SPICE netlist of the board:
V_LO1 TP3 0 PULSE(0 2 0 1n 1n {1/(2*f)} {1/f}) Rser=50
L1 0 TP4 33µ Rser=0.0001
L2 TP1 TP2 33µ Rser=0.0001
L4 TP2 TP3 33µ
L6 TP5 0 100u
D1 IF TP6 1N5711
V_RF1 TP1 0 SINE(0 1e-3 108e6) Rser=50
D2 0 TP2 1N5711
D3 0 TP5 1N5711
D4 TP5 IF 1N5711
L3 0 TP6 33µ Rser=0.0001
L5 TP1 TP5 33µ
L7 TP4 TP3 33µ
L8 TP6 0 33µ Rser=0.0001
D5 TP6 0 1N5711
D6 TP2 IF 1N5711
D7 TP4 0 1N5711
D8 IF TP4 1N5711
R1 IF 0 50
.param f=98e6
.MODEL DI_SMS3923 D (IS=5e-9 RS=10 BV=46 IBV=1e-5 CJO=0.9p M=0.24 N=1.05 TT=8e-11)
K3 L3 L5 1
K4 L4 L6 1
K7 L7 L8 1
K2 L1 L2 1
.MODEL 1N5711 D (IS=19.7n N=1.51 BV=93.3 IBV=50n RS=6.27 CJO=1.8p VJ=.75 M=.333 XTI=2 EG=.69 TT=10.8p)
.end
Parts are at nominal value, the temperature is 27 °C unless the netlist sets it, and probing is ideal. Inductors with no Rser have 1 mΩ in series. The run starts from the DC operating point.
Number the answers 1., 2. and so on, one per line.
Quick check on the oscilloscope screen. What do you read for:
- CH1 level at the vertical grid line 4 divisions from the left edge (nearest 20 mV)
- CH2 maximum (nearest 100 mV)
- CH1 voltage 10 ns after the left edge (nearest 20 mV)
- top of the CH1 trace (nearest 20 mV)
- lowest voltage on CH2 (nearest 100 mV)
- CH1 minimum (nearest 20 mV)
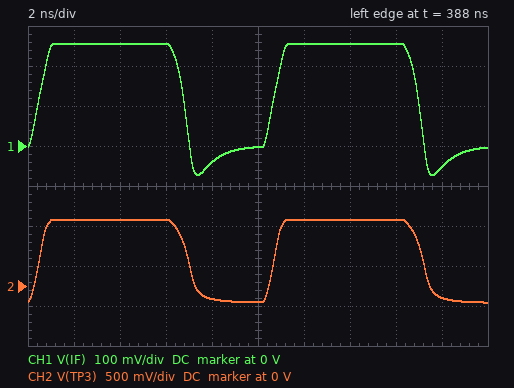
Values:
1. -40 mV
2. 800 mV
3. 0 V
4. 260 mV
5. -200 mV
6. -80 mV
